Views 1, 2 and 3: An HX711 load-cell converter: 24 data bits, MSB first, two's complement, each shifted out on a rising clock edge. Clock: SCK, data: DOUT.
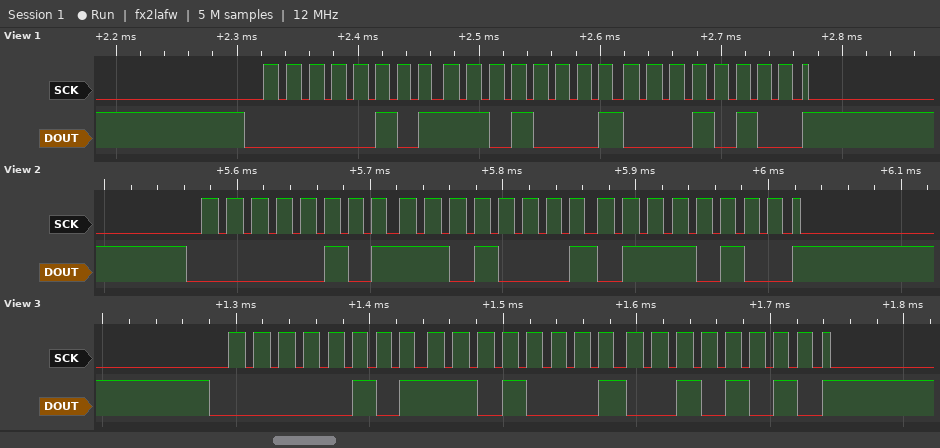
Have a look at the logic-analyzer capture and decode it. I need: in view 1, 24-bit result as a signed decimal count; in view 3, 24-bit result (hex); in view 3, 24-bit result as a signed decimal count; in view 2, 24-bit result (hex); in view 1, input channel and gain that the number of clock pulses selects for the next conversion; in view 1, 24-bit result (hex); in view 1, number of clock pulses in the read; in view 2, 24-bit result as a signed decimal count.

381204
0x05D12A
381226
0x05D174
channel A, gain 128
0x05D114
25
381300
